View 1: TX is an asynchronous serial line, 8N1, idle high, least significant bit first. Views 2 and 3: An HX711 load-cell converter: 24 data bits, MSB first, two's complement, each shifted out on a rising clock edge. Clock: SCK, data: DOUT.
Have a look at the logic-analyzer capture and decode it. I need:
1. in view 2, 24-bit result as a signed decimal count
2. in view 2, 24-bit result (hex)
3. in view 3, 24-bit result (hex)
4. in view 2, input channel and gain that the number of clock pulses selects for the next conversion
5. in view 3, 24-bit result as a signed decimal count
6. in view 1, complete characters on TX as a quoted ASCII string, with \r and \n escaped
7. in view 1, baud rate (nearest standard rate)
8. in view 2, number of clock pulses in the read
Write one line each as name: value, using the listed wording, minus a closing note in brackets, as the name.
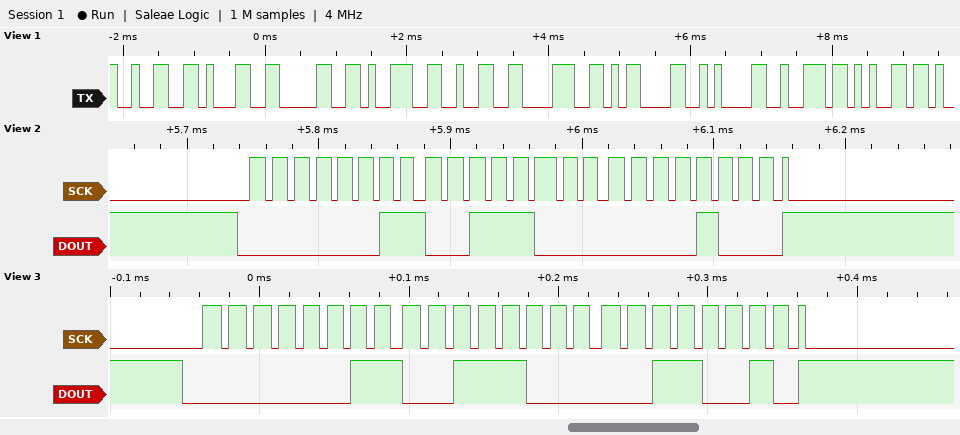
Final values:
in view 2, 24-bit result as a signed decimal count: 210952
in view 2, 24-bit result: 0x033808
in view 3, 24-bit result: 0x033832
in view 2, input channel and gain that the number of clock pulses selects for the next conversion: channel A, gain 128
in view 3, 24-bit result as a signed decimal count: 210994
in view 1, complete characters on TX as a quoted ASCII string, with \r and \n escaped: "210928\r\nre"
in view 1, baud rate: 9600 baud
in view 2, number of clock pulses in the read: 25
